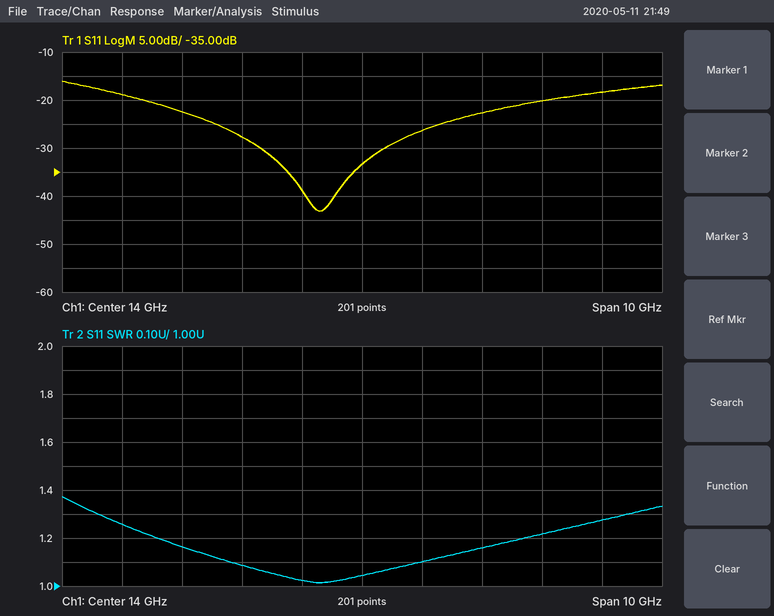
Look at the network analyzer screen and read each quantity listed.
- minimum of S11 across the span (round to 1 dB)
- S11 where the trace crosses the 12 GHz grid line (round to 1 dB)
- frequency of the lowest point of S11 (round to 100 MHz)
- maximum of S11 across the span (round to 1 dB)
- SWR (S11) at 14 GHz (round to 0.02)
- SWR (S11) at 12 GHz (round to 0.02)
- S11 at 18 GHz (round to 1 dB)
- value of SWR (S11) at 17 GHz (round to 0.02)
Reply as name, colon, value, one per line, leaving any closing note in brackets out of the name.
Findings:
minimum of S11 across the span: -43 dB
S11 where the trace crosses the 12 GHz grid line: -28 dB
frequency of the lowest point of S11: 13.3 GHz
maximum of S11 across the span: -16 dB
SWR (S11) at 14 GHz: 1.04
SWR (S11) at 12 GHz: 1.08
S11 at 18 GHz: -18 dB
value of SWR (S11) at 17 GHz: 1.22
